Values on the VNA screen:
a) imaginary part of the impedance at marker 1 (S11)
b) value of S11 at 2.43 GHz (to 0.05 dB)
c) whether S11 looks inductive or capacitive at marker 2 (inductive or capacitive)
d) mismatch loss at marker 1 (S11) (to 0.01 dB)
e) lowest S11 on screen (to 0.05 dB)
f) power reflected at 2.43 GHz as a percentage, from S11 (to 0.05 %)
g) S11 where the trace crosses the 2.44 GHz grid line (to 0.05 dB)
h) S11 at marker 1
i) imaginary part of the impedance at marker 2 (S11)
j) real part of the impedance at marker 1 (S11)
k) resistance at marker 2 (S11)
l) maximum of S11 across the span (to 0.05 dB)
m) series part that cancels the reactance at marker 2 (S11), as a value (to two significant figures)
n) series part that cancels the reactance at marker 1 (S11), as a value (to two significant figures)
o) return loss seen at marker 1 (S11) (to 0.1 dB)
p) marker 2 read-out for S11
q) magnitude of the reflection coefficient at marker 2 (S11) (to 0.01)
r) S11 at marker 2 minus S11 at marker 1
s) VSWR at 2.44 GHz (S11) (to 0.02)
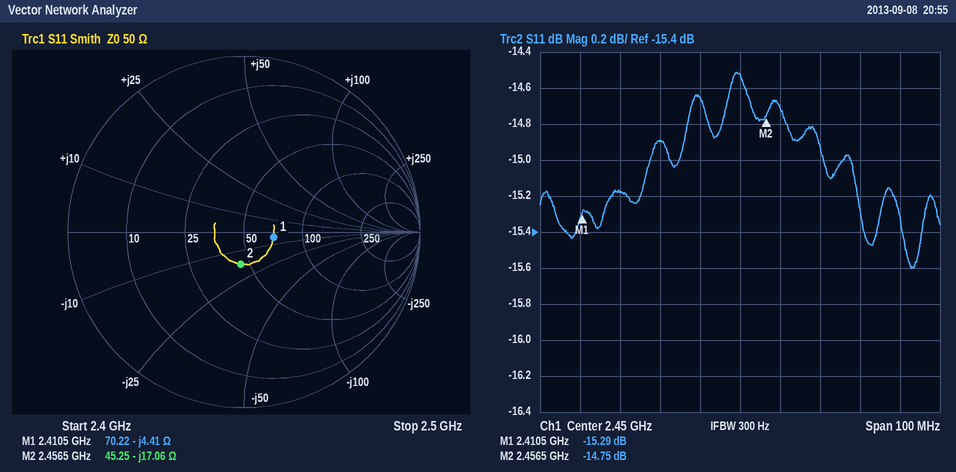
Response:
-4.41 Ω
-14.90 dB
capacitive
0.13 dB
-15.60 dB
3.25 %
-14.65 dB
-15.29 dB
-17.06 Ω
70.22 Ω
45.25 Ω
-14.50 dB
1.1 nH
290 pH
15.3 dB
-14.75 dB
0.18
0.54 dB
1.46
